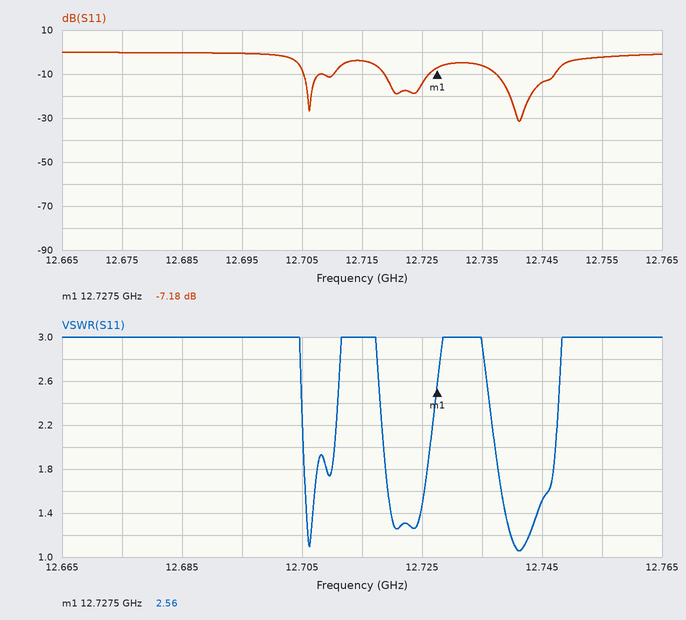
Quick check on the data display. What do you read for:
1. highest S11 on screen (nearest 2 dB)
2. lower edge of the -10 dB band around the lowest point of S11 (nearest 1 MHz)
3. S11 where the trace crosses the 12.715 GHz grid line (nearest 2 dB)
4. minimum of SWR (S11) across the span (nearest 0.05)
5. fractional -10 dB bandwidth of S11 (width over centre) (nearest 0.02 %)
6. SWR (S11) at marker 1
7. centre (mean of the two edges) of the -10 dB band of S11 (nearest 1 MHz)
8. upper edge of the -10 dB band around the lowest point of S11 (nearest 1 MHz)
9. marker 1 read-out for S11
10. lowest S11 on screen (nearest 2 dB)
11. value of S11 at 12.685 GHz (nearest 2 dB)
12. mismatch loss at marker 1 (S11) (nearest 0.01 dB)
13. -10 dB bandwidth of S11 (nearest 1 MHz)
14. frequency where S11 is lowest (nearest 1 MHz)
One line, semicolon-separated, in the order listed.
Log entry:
0 dB; 12.737 GHz; -4 dB; 1.05; 0.08 %; 2.56; 12.742 GHz; 12.747 GHz; -7.18 dB; -32 dB; 0 dB; 0.92 dB; 10 MHz; 12.741 GHz
